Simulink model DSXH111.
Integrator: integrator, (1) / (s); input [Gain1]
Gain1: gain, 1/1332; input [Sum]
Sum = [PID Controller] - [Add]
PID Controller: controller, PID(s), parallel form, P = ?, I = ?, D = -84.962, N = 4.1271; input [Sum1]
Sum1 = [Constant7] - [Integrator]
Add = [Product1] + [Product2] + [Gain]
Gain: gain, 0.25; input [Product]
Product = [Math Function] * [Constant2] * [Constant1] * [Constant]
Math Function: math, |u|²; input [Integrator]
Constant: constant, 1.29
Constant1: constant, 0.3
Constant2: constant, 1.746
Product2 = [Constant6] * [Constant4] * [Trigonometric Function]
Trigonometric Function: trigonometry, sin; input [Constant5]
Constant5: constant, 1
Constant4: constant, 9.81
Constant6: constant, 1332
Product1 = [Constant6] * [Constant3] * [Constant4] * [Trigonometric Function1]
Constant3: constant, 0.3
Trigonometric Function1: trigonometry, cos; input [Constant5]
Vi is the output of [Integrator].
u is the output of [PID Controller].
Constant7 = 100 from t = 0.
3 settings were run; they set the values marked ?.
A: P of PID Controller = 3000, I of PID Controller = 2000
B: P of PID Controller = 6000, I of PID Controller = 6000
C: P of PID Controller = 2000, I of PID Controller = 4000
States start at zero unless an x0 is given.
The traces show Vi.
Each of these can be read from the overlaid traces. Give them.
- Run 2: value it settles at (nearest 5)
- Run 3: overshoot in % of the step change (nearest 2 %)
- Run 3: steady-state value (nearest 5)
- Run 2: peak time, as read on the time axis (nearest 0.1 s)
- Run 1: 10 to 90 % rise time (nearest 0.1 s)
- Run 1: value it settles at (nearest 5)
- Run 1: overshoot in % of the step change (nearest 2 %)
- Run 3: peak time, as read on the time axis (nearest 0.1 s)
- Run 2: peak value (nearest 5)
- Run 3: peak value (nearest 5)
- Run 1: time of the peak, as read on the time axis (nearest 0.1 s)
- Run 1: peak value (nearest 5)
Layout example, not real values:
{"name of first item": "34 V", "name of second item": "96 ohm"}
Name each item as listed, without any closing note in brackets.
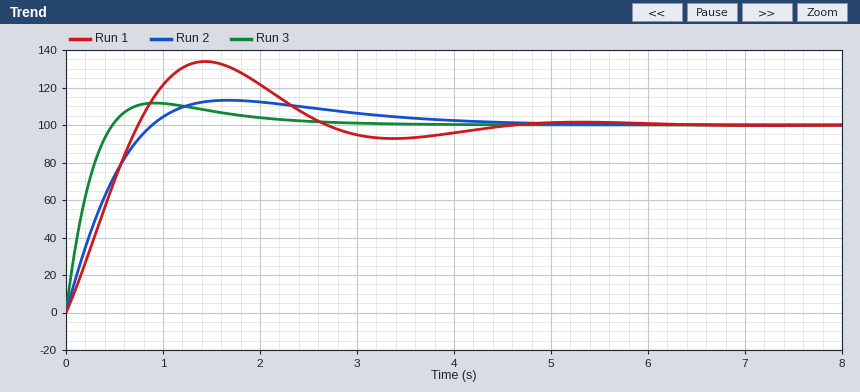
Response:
{"Run 2: value it settles at": "100", "Run 3: overshoot in % of the step change": "12 %", "Run 3: steady-state value": "100", "Run 2: peak time, as read on the time axis": "1.7 s", "Run 1: 10 to 90 % rise time": "0.6 s", "Run 1: value it settles at": "100", "Run 1: overshoot in % of the step change": "34 %", "Run 3: peak time, as read on the time axis": "0.9 s", "Run 2: peak value": "115", "Run 3: peak value": "110", "Run 1: time of the peak, as read on the time axis": "1.4 s", "Run 1: peak value": "135"}
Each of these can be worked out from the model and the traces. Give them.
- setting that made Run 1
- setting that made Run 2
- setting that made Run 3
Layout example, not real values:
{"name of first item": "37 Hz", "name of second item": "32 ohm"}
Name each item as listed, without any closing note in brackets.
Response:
{"setting that made Run 1": "C", "setting that made Run 2": "A", "setting that made Run 3": "B"}
